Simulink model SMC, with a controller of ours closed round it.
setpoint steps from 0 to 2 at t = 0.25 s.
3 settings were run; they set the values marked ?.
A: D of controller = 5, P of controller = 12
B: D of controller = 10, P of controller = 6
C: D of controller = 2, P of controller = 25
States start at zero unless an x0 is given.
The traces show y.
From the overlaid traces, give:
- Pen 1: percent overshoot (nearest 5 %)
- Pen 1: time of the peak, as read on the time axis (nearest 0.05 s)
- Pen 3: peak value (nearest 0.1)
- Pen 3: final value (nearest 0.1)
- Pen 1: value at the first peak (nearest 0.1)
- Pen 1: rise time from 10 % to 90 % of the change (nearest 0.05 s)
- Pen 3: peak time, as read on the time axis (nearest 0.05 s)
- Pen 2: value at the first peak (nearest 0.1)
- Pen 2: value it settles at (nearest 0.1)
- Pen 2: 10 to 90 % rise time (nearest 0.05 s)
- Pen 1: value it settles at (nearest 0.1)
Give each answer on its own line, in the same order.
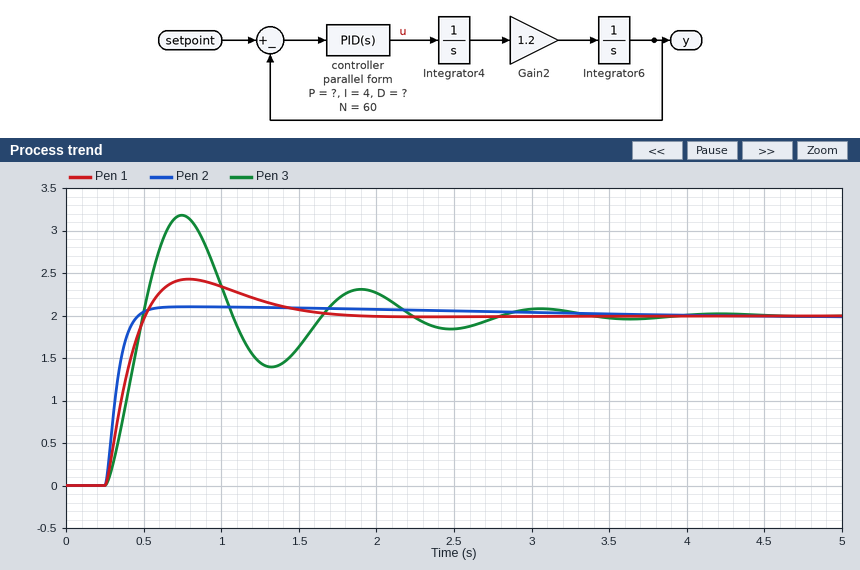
20 %
0.80 s
3.2
2.0
2.4
0.20 s
0.75 s
2.1
2.0
0.15 s
2.0
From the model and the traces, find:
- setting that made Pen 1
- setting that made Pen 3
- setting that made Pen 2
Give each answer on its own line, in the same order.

A
C
B
